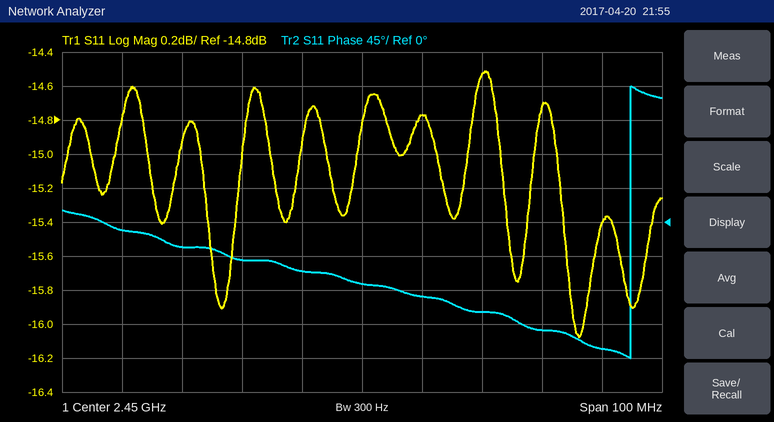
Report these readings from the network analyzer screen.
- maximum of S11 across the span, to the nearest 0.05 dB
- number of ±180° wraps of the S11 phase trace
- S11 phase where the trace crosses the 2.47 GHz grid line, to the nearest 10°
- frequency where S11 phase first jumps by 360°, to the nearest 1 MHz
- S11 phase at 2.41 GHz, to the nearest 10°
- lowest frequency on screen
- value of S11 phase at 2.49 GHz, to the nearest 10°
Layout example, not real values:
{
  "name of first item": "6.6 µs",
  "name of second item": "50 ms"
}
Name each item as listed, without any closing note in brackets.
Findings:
{
  "maximum of S11 across the span, to the nearest 0.05 dB": "-14.50 dB",
  "number of ±180° wraps of the S11 phase trace": "1",
  "S11 phase where the trace crosses the 2.47 GHz grid line, to the nearest 10°": "-120°",
  "frequency where S11 phase first jumps by 360°, to the nearest 1 MHz": "2.495 GHz",
  "S11 phase at 2.41 GHz, to the nearest 10°": "-10°",
  "lowest frequency on screen": "2.4 GHz",
  "value of S11 phase at 2.49 GHz, to the nearest 10°": "-170°"
}
